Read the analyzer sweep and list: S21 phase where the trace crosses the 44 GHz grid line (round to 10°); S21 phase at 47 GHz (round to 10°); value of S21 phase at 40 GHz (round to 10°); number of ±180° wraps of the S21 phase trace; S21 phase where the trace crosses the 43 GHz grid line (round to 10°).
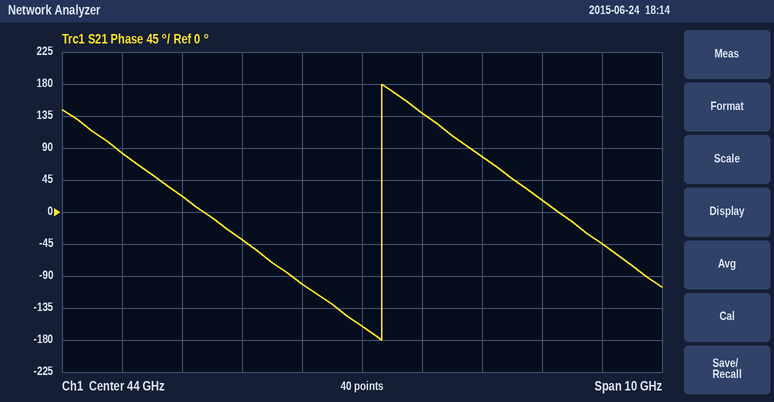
-160°
20°
80°
1
-100°
